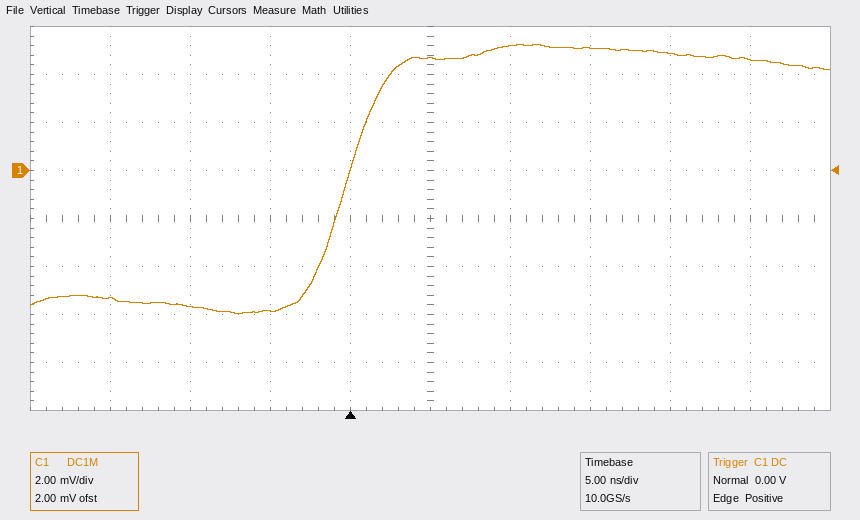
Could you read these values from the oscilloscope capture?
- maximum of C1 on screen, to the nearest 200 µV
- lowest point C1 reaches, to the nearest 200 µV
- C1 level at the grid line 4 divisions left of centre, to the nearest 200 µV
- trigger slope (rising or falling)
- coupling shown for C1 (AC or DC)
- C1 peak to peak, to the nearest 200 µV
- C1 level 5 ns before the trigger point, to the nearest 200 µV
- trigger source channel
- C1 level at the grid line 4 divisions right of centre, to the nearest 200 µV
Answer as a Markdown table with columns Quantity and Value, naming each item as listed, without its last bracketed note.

| Quantity | Value |
|---|---|
| maximum of C1 on screen, to the nearest 200 µV | 5.2 mV |
| lowest point C1 reaches, to the nearest 200 µV | -6.0 mV |
| C1 level at the grid line 4 divisions left of centre, to the nearest 200 µV | -5.4 mV |
| trigger slope | rising |
| coupling shown for C1 | DC |
| C1 peak to peak, to the nearest 200 µV | 11.2 mV |
| C1 level 5 ns before the trigger point, to the nearest 200 µV | -5.8 mV |
| trigger source channel | C1 |
| C1 level at the grid line 4 divisions right of centre, to the nearest 200 µV | 4.6 mV |
